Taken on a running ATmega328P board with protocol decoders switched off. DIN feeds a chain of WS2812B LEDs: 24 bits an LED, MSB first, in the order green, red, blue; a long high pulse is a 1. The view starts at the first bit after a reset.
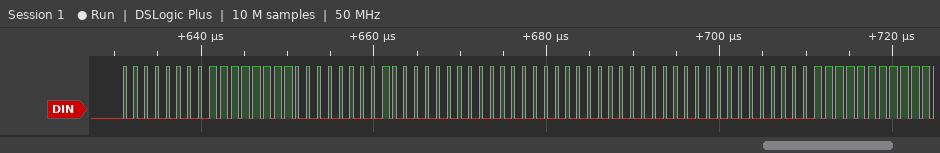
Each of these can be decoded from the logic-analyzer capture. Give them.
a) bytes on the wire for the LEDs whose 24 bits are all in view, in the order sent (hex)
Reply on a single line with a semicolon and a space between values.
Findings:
00 FF 00 80 00 00 00 00 FF
